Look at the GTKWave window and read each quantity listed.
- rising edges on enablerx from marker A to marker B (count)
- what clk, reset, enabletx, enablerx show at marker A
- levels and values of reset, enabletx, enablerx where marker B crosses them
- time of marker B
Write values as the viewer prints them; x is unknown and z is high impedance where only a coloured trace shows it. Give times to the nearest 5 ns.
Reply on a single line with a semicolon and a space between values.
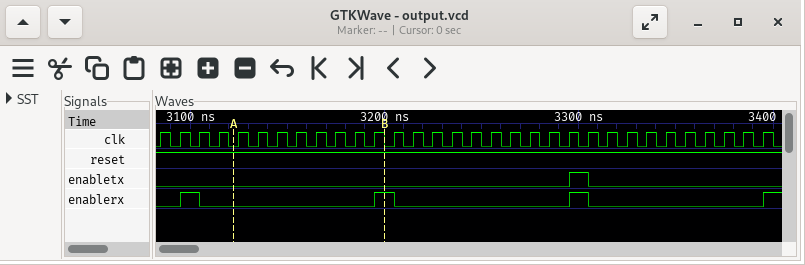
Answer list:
1; clk=0, reset=1, enabletx=0, enablerx=0; reset=1, enabletx=0, enablerx=1; 3200 ns
